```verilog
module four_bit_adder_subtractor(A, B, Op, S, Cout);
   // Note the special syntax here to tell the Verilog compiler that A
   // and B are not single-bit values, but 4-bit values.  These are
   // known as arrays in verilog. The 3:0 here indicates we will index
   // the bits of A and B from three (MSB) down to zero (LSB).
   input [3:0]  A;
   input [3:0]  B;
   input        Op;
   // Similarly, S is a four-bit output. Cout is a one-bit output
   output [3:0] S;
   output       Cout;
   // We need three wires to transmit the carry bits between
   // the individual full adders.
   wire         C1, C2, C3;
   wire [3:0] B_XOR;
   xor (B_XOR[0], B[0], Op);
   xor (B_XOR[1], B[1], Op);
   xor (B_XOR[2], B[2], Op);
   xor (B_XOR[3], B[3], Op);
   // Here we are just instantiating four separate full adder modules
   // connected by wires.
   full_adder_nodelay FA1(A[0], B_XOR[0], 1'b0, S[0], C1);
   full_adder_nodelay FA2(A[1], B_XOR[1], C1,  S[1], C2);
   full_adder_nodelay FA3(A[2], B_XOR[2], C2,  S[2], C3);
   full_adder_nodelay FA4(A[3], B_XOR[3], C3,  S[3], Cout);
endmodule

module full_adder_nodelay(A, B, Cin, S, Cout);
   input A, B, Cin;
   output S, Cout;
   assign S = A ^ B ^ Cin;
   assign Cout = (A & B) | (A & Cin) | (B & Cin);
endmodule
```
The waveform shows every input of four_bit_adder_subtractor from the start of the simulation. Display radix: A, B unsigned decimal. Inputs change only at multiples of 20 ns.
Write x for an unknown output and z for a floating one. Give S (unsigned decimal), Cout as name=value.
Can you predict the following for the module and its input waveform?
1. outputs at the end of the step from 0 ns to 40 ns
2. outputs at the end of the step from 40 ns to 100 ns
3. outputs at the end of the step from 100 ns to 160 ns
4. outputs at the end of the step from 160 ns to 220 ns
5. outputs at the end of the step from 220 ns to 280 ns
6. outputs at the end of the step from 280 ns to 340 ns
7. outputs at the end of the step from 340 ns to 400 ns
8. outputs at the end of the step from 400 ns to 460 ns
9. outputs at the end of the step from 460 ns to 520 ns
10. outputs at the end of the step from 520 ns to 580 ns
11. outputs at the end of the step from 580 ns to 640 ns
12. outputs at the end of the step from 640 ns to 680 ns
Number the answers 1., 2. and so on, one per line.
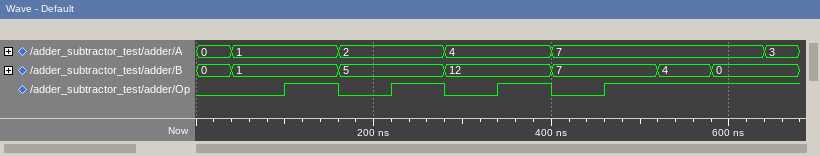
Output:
1. S=0, Cout=0
2. S=2, Cout=0
3. S=15, Cout=0
4. S=7, Cout=0
5. S=12, Cout=0
6. S=0, Cout=1
7. S=7, Cout=0
8. S=14, Cout=0
9. S=15, Cout=0
10. S=2, Cout=1
11. S=6, Cout=1
12. S=2, Cout=1
